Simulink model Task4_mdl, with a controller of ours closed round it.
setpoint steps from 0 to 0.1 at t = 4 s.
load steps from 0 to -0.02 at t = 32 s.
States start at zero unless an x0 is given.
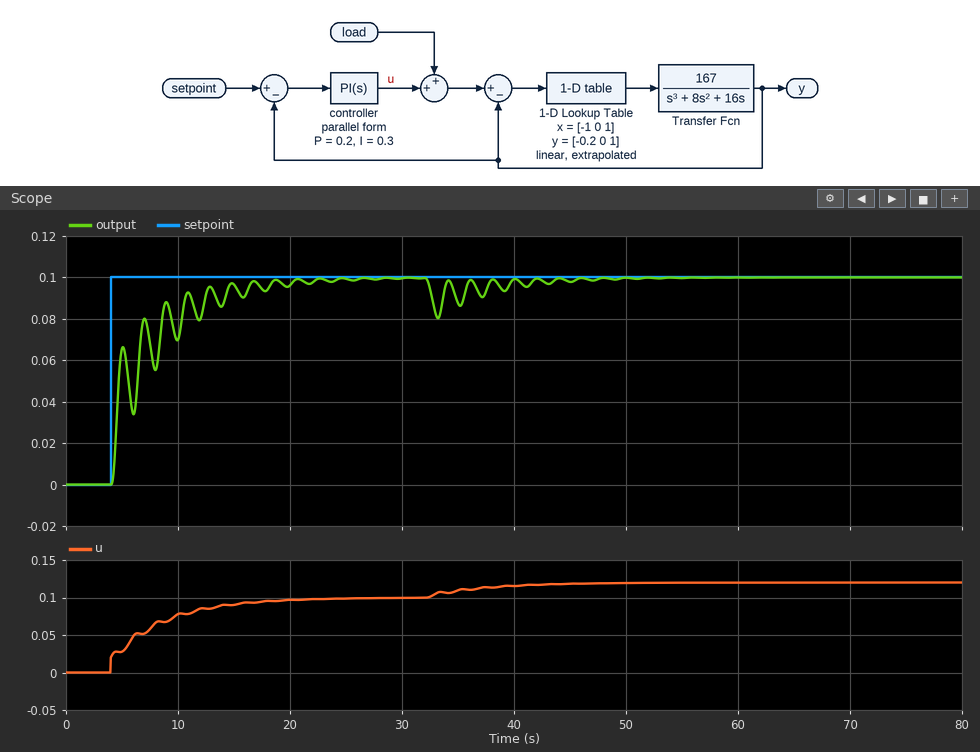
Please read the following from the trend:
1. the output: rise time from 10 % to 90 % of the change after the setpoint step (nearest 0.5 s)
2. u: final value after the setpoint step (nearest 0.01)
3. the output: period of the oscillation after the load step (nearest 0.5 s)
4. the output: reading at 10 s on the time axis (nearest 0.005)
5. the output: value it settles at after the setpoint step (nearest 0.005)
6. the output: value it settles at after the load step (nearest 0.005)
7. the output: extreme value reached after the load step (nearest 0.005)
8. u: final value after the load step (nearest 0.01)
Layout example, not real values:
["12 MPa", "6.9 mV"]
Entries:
["6.5 s", "0.10", "2.0 s", "0.070", "0.100", "0.100", "0.080", "0.12"]
